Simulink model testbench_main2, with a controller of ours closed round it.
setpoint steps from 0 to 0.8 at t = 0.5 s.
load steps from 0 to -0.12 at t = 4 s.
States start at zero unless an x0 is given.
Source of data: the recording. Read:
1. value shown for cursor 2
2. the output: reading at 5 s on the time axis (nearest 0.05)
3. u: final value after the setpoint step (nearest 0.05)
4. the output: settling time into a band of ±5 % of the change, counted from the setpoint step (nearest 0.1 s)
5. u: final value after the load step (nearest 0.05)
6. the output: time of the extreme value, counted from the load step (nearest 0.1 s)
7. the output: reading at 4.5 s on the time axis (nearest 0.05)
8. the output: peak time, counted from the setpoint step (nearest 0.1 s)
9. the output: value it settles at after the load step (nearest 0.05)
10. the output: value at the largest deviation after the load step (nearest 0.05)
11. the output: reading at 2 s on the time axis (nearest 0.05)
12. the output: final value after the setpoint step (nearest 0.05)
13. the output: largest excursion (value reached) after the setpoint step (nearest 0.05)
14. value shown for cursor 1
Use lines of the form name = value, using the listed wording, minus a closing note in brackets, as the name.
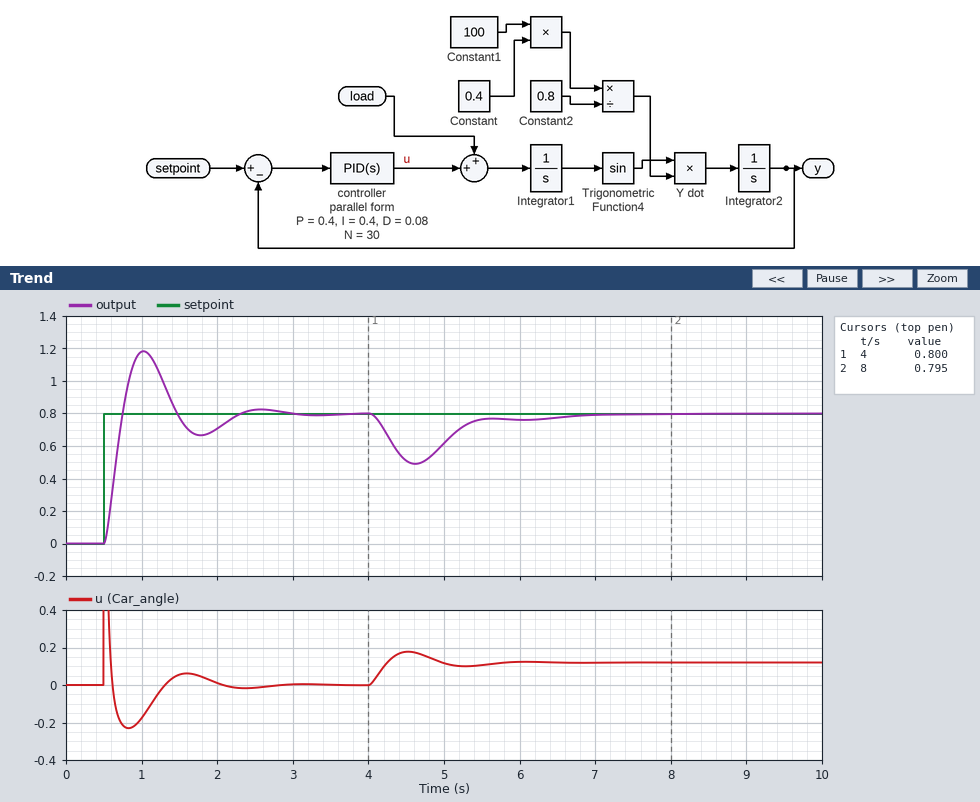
value shown for cursor 2 = 0.795
the output: reading at 5 s on the time axis = 0.60
u: final value after the setpoint step = 0.00
the output: settling time into a band of ±5 % of the change, counted from the setpoint step = 1.7 s
u: final value after the load step = 0.10
the output: time of the extreme value, counted from the load step = 0.6 s
the output: reading at 4.5 s on the time axis = 0.50
the output: peak time, counted from the setpoint step = 0.5 s
the output: value it settles at after the load step = 0.80
the output: value at the largest deviation after the load step = 0.50
the output: reading at 2 s on the time axis = 0.70
the output: final value after the setpoint step = 0.80
the output: largest excursion (value reached) after the setpoint step = 1.20
value shown for cursor 1 = 0.800
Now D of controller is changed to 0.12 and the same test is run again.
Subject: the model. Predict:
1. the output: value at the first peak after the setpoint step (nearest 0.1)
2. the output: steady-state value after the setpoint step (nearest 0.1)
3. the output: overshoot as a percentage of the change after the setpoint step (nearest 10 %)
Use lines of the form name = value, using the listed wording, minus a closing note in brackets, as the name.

the output: value at the first peak after the setpoint step = 1.1
the output: steady-state value after the setpoint step = 0.8
the output: overshoot as a percentage of the change after the setpoint step = 30 %
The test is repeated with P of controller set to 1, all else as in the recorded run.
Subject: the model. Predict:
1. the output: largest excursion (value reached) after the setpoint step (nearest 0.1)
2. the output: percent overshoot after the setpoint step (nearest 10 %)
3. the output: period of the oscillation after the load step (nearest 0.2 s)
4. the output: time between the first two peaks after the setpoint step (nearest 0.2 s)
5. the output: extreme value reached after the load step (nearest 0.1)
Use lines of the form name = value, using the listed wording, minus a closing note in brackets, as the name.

the output: largest excursion (value reached) after the setpoint step = 1.3
the output: percent overshoot after the setpoint step = 60 %
the output: period of the oscillation after the load step = 0.8 s
the output: time between the first two peaks after the setpoint step = 0.8 s
the output: extreme value reached after the load step = 0.6
